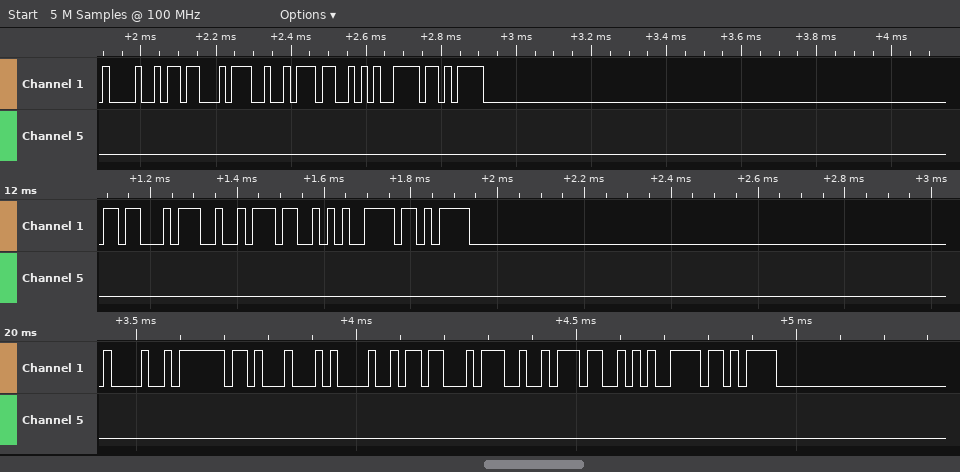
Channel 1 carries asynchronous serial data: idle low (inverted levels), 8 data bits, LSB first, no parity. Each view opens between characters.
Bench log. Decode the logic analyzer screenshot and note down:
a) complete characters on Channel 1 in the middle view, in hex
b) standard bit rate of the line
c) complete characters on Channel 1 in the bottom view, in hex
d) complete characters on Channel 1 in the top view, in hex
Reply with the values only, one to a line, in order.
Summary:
72, 6C, 64, 0D, 0A
57600 baud
6F, 20, 77, 6F, 72, 6C, 64, 0D, 0A
6F, 72, 6C, 64, 0D, 0A
